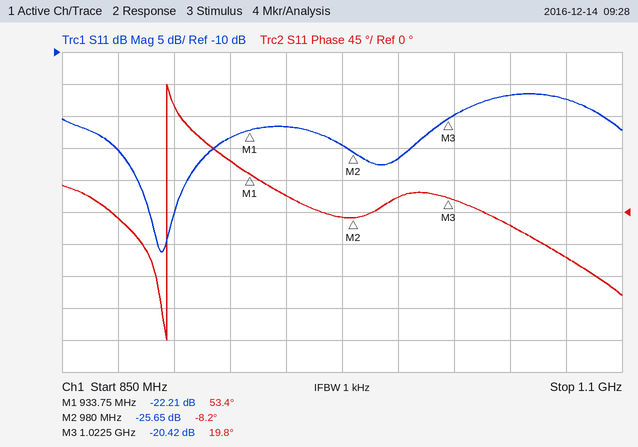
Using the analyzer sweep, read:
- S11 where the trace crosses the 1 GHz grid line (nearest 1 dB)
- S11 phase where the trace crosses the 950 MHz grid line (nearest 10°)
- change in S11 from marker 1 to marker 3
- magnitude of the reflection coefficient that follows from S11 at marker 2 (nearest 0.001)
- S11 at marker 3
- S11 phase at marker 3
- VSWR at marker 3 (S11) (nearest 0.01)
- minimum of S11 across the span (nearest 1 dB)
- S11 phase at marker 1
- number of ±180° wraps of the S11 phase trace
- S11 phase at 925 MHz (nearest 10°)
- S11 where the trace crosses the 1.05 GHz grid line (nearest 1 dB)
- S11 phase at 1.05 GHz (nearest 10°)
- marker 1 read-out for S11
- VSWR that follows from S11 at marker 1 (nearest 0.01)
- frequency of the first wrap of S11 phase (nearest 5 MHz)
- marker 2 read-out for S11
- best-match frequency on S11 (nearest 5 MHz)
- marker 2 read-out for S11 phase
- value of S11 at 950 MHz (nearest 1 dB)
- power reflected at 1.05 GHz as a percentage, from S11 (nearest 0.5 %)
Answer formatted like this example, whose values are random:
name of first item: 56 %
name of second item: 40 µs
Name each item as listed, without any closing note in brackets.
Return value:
S11 where the trace crosses the 1 GHz grid line: -27 dB
S11 phase where the trace crosses the 950 MHz grid line: 20°
change in S11 from marker 1 to marker 3: 1.79 dB
magnitude of the reflection coefficient that follows from S11 at marker 2: 0.052
S11 at marker 3: -20.42 dB
S11 phase at marker 3: 19.8°
VSWR at marker 3 (S11): 1.21
minimum of S11 across the span: -41 dB
S11 phase at marker 1: 53.4°
number of ±180° wraps of the S11 phase trace: 1
S11 phase at 925 MHz: 70°
S11 where the trace crosses the 1.05 GHz grid line: -17 dB
S11 phase at 1.05 GHz: -20°
marker 1 read-out for S11: -22.21 dB
VSWR that follows from S11 at marker 1: 1.17
frequency of the first wrap of S11 phase: 895 MHz
marker 2 read-out for S11: -25.65 dB
best-match frequency on S11: 895 MHz
marker 2 read-out for S11 phase: -8.2°
value of S11 at 950 MHz: -22 dB
power reflected at 1.05 GHz as a percentage, from S11: 2.0 %
